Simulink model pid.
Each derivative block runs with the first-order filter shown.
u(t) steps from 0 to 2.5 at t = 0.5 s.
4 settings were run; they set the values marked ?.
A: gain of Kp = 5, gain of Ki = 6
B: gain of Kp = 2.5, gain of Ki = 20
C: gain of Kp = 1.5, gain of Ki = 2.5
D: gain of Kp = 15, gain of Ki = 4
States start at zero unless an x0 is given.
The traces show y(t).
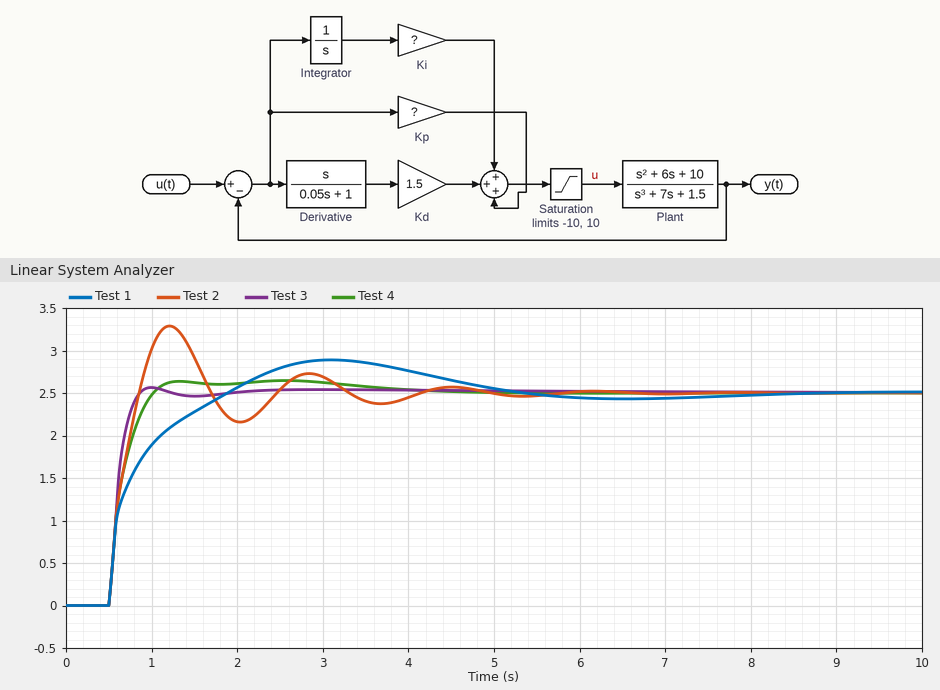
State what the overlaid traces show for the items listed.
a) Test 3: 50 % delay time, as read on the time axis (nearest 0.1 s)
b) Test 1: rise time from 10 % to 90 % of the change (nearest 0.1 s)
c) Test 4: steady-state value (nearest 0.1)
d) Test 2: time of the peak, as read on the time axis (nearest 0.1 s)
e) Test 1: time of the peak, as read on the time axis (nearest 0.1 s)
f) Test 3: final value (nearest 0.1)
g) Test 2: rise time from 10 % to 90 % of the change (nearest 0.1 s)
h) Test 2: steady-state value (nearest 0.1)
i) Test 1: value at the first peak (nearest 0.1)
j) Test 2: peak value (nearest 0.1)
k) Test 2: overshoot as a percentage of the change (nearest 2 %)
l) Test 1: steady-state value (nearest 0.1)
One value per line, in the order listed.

0.6 s
0.9 s
2.5
1.2 s
3.1 s
2.5
0.3 s
2.5
2.9
3.3
32 %
2.5
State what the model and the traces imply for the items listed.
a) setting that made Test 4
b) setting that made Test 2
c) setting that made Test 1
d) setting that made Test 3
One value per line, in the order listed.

A
B
C
D
